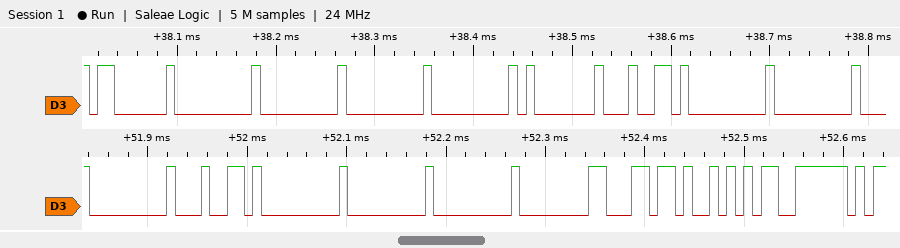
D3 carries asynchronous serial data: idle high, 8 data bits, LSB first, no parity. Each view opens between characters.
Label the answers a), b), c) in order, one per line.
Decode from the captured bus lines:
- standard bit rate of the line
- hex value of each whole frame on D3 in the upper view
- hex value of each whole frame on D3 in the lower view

a) 115200 baud
b) 03, 00, 00, 00, 00, 01, 64, 00, 00
c) 00, 64, 00, 00, 00, 80, 6C, AA, 7E
